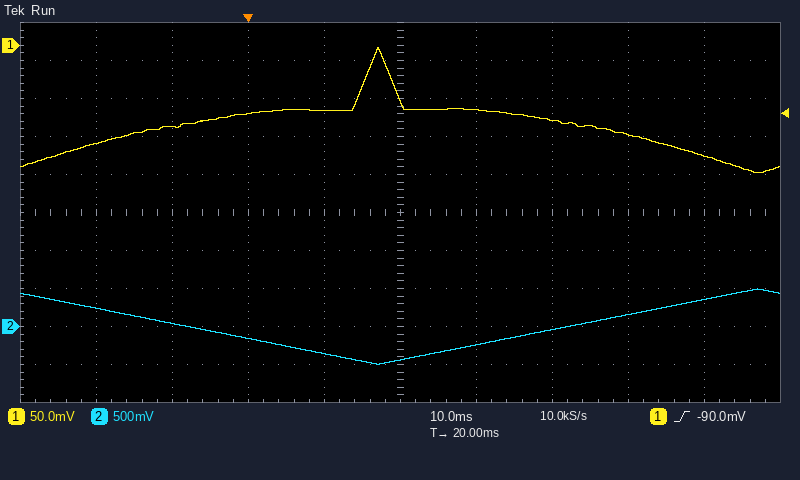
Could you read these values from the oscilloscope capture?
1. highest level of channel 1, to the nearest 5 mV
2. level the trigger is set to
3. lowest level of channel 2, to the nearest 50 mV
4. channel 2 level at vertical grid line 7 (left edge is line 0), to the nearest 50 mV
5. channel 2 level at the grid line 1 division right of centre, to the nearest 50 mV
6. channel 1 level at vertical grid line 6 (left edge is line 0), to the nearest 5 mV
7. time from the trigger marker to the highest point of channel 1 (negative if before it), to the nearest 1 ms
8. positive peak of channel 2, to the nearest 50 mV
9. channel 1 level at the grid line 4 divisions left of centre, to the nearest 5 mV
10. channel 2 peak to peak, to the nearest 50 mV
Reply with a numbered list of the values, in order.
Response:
1. -5 mV
2. -90.0 mV
3. -500 mV
4. -50 mV
5. -250 mV
6. -85 mV
7. +17 ms
8. 500 mV
9. -130 mV
10. 1.00 V
